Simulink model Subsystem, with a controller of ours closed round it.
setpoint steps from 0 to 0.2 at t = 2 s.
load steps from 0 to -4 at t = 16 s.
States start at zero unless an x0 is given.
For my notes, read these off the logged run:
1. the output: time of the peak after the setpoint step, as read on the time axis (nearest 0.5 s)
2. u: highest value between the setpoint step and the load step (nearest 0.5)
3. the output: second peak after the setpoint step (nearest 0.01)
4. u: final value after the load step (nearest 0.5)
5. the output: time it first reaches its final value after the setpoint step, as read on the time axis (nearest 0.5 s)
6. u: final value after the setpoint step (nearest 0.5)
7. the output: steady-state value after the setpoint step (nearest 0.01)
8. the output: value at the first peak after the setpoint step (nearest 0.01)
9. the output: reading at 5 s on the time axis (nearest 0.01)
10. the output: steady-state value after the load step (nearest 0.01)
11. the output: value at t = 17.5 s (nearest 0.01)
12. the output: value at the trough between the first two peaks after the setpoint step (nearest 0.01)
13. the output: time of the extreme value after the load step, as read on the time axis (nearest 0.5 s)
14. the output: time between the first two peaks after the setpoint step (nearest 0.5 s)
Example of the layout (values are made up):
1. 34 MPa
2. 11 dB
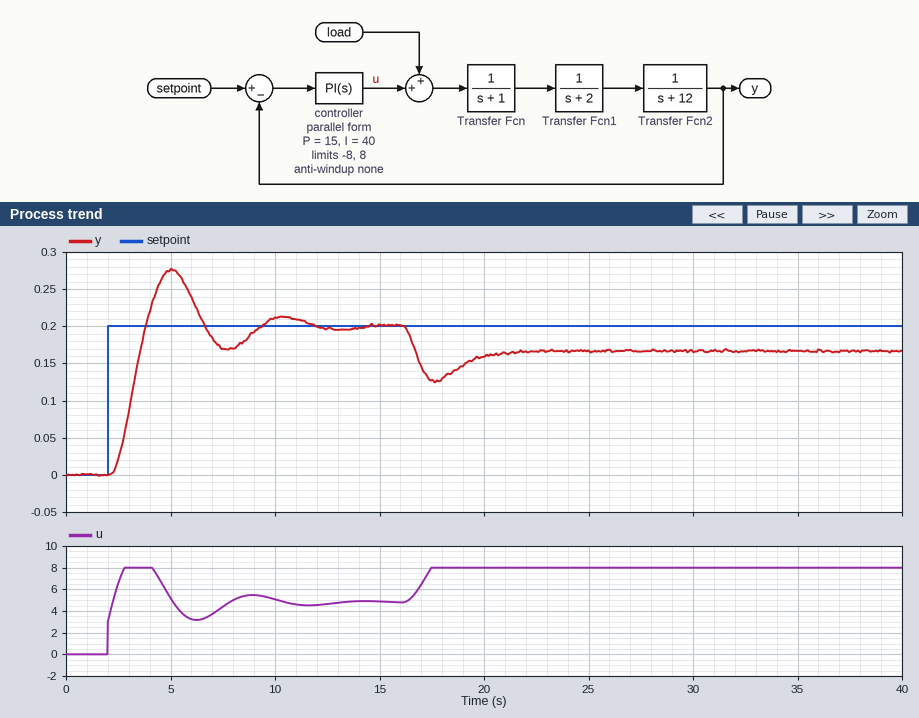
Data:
1. 5.0 s
2. 8.0
3. 0.21
4. 8.0
5. 4.0 s
6. 5.0
7. 0.20
8. 0.28
9. 0.28
10. 0.17
11. 0.13
12. 0.17
13. 17.5 s
14. 5.5 s
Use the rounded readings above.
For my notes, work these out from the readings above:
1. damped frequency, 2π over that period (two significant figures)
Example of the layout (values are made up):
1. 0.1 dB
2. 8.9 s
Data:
1. 1.1 rad/s
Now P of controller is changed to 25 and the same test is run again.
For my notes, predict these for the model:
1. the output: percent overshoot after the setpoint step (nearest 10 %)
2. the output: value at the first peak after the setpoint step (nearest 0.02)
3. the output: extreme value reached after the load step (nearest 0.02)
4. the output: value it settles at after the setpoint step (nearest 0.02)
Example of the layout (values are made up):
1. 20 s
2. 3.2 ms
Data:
1. 30 %
2. 0.26
3. 0.14
4. 0.20
